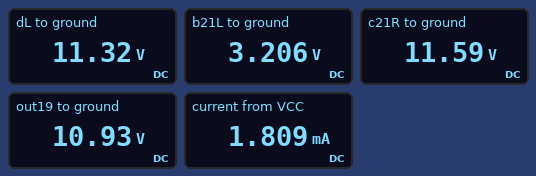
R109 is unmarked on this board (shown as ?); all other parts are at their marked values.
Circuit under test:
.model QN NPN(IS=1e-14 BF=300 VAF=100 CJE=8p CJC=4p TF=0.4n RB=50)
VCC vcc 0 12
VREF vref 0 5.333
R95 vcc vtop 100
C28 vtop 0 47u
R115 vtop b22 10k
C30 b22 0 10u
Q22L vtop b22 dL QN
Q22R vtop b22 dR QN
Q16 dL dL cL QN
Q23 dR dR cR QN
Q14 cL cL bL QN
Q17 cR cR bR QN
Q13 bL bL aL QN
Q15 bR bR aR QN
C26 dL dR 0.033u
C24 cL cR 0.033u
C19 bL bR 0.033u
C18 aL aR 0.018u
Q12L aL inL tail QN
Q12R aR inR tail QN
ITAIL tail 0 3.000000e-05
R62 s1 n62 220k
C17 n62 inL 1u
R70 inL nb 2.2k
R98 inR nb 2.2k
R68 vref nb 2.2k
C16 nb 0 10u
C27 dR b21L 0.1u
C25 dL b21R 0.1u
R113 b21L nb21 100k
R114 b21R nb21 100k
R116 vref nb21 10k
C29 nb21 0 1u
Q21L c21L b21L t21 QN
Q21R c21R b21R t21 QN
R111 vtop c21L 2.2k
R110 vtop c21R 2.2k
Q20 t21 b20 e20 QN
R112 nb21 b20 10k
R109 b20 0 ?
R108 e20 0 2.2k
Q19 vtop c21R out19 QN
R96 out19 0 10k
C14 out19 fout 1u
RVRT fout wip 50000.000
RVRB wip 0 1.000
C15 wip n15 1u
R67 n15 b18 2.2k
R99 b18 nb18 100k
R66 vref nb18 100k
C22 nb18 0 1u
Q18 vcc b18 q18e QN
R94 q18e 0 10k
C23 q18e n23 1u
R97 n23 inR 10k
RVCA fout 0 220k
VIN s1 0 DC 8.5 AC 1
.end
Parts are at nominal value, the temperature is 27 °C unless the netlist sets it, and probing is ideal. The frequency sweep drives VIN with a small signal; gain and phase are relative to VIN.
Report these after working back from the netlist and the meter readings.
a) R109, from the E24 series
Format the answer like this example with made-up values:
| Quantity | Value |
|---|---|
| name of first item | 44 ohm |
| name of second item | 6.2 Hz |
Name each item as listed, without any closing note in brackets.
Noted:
| Quantity | Value |
|---|---|
| R109, from the E24 series | 5.6 kΩ |
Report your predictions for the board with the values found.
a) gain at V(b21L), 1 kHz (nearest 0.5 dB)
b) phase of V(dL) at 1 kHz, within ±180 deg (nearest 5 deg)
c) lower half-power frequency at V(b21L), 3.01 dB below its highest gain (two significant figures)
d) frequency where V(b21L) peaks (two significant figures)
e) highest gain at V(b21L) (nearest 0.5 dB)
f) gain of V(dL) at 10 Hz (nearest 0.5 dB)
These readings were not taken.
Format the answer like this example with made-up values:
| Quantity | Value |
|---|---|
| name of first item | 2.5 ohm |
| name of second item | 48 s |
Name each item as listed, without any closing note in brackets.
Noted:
| Quantity | Value |
|---|---|
| gain at V(b21L), 1 kHz | -62.0 dB |
| phase of V(dL) at 1 kHz, within ±180 deg | 45 deg |
| lower half-power frequency at V(b21L), 3.01 dB below its highest gain | 27 Hz |
| frequency where V(b21L) peaks | 87 Hz |
| highest gain at V(b21L) | -48.0 dB |
| gain of V(dL) at 10 Hz | -45.5 dB |
